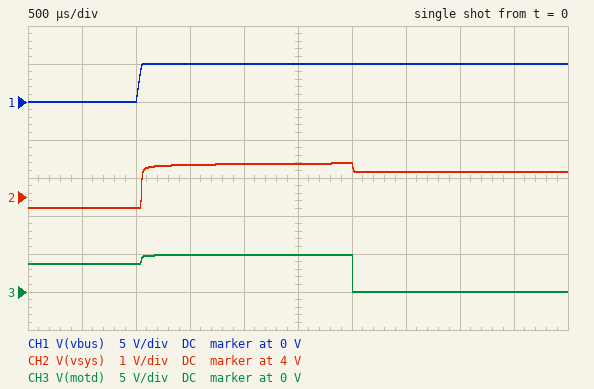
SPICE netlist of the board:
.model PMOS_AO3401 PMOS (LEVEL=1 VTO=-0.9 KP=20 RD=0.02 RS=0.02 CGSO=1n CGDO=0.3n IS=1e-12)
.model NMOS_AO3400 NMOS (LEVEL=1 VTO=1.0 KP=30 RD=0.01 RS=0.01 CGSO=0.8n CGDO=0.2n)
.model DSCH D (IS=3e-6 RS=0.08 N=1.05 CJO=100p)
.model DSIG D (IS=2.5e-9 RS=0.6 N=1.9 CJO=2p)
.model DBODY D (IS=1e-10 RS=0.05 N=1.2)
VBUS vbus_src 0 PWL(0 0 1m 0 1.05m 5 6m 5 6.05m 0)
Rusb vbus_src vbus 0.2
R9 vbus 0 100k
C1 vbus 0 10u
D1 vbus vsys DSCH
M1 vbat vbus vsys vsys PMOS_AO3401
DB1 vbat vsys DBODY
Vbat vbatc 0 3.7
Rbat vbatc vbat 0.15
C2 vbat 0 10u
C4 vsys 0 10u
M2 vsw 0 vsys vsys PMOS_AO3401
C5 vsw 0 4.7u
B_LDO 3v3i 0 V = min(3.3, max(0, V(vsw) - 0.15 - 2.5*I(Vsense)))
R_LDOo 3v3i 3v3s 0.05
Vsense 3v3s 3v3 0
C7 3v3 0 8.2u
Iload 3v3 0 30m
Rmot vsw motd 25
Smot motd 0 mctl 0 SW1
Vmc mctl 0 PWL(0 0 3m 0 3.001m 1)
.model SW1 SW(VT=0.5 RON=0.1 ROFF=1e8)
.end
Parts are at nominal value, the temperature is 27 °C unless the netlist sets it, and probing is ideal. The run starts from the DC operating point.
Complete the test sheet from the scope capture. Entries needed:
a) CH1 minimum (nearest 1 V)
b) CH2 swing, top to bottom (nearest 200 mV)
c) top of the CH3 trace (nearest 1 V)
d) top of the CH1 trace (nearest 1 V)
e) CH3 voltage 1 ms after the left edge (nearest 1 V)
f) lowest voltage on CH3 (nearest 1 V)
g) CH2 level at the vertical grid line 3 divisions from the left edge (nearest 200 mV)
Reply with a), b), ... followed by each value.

a) 0 V
b) 1.2 V
c) 5 V
d) 5 V
e) 4 V
f) 0 V
g) 4.8 V
